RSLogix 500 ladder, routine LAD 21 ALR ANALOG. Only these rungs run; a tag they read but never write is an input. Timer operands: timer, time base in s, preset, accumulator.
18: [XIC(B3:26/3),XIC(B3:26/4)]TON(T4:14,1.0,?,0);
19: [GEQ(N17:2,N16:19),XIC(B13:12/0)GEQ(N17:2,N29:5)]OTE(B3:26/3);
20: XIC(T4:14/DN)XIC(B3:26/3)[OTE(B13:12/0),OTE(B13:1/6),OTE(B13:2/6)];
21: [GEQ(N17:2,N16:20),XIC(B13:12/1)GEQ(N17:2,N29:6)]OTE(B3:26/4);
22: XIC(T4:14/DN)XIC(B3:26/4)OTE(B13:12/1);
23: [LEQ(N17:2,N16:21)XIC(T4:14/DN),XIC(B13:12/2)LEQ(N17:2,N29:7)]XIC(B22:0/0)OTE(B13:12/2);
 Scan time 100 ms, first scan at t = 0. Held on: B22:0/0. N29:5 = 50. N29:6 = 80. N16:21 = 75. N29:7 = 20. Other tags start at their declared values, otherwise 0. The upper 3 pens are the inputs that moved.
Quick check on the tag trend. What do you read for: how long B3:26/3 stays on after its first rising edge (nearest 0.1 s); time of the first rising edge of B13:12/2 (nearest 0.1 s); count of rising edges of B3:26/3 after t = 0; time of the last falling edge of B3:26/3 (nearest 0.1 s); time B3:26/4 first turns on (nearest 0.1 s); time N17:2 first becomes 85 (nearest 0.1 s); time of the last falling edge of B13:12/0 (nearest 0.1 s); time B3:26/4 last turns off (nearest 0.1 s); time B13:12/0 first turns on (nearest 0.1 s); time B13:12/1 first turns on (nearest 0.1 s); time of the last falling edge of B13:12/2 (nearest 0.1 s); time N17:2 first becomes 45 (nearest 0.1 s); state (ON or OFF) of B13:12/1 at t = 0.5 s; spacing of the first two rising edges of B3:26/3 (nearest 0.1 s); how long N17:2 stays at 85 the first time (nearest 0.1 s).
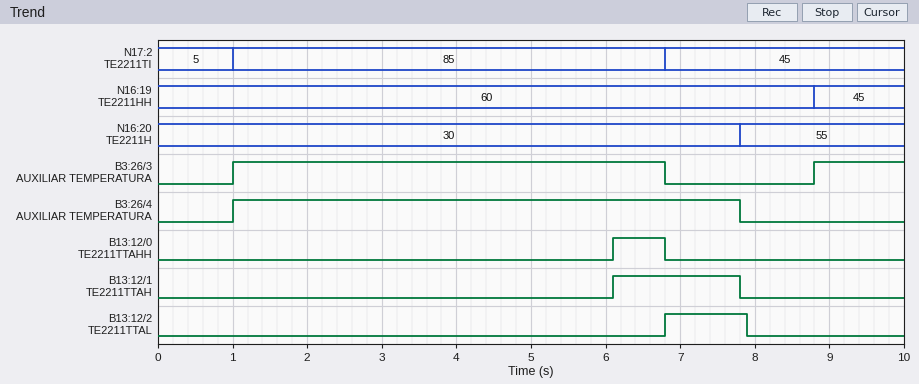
5.8 s
6.8 s
2
6.8 s
1.0 s
1.0 s
6.8 s
7.8 s
6.1 s
6.1 s
7.9 s
6.8 s
OFF
7.8 s
5.8 s
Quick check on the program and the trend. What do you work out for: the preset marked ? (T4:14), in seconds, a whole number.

5 s
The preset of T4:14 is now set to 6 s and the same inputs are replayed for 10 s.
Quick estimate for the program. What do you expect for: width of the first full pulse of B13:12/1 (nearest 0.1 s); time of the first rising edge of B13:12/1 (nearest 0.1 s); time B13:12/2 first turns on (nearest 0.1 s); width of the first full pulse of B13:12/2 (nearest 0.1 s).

0.7 s
7.1 s
7.1 s
0.8 s
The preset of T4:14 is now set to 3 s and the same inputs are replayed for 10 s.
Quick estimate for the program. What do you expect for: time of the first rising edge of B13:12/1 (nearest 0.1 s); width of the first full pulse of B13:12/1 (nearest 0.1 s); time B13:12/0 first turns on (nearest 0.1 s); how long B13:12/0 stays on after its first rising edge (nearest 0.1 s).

4.1 s
3.7 s
4.1 s
2.7 s
